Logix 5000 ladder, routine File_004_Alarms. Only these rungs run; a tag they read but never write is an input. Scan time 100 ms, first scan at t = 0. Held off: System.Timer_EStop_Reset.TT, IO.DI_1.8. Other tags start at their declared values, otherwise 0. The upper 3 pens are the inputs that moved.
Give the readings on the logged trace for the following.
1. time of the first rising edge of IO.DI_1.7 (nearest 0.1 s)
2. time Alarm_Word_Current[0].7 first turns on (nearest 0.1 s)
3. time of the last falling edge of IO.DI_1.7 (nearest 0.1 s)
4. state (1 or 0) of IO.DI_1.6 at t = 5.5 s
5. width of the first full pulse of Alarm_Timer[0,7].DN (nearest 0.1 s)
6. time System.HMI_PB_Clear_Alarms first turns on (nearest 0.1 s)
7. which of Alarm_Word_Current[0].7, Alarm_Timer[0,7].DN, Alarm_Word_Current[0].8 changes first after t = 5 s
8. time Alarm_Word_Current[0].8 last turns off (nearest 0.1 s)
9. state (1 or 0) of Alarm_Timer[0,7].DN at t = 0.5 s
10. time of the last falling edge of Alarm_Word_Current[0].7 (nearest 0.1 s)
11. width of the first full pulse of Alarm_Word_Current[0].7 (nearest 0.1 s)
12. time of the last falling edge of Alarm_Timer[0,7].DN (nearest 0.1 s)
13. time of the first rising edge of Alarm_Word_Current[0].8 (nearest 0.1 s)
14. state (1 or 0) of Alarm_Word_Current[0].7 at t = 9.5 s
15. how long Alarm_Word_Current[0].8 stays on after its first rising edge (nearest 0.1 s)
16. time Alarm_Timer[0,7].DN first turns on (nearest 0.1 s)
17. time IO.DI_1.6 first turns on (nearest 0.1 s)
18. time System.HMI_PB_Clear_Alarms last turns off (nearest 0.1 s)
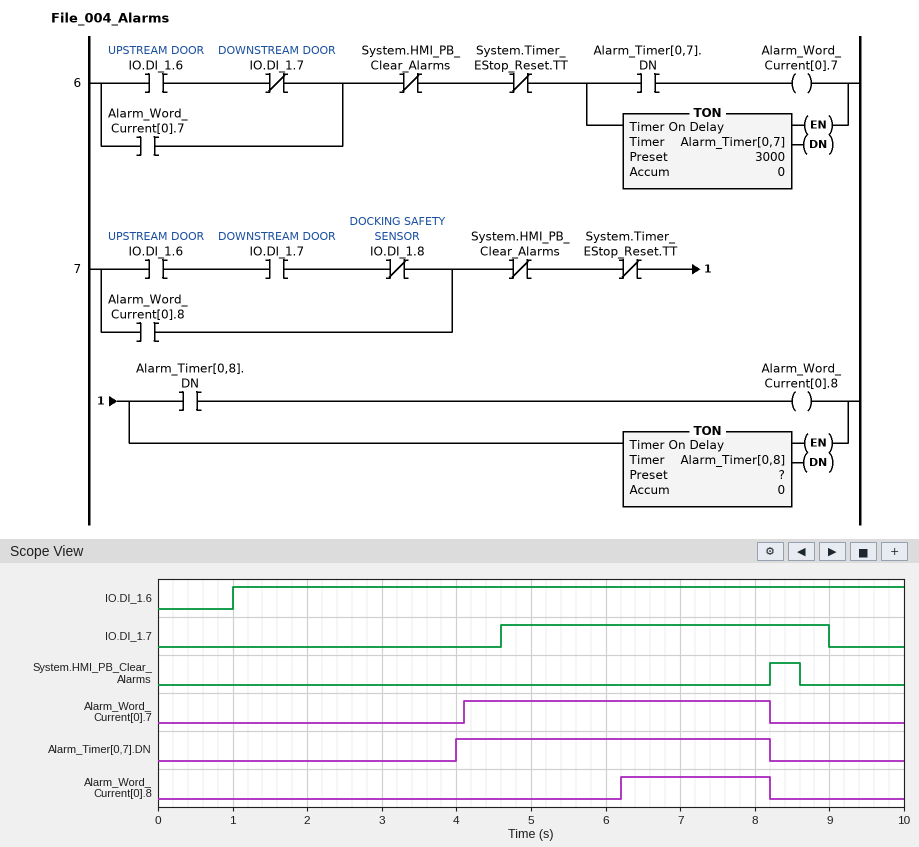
4.6 s
4.1 s
9.0 s
1
4.2 s
8.2 s
Alarm_Word_Current[0].8
8.2 s
0
8.2 s
4.1 s
8.2 s
6.2 s
0
2.0 s
4.0 s
1.0 s
8.6 s
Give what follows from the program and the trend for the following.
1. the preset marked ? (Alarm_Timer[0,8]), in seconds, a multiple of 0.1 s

1.5 s
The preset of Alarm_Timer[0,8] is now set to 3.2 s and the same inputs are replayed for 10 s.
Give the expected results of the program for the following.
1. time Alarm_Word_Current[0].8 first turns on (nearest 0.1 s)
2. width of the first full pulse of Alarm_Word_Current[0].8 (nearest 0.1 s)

7.9 s
0.3 s
